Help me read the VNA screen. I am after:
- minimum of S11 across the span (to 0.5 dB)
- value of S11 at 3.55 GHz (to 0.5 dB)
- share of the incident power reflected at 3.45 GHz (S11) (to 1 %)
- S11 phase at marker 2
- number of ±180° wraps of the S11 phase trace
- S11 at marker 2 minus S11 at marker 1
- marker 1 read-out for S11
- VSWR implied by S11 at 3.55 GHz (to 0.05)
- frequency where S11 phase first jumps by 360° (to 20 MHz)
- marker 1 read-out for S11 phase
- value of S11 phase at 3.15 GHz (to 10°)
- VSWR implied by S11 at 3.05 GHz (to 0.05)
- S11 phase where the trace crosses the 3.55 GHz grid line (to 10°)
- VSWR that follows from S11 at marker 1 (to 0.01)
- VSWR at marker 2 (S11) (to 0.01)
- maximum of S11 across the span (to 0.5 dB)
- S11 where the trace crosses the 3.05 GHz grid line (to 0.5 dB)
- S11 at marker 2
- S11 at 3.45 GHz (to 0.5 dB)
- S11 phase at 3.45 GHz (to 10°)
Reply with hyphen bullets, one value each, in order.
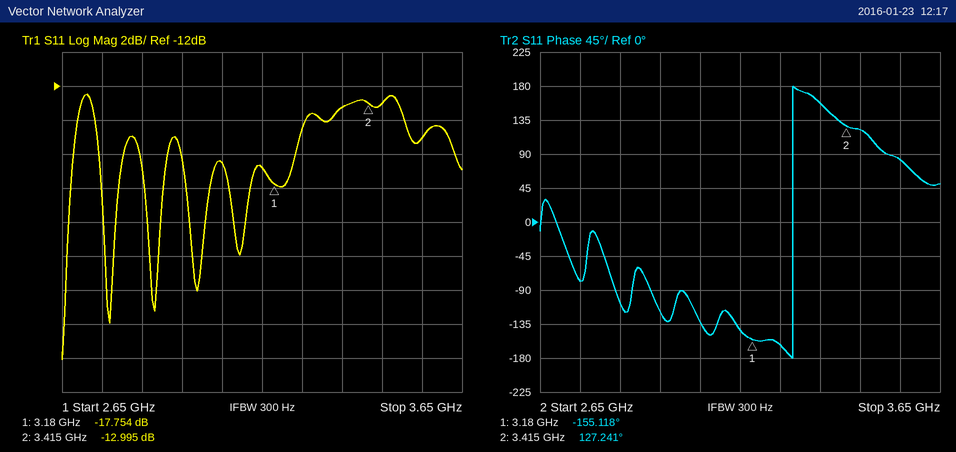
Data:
- -28.0 dB
- -15.0 dB
- 5 %
- 127.241°
- 1
- 4.759 dB
- -17.754 dB
- 1.45
- 3.28 GHz
- -155.118°
- -140°
- 1.35
- 80°
- 1.30
- 1.58
- -12.5 dB
- -16.5 dB
- -12.995 dB
- -13.0 dB
- 120°
